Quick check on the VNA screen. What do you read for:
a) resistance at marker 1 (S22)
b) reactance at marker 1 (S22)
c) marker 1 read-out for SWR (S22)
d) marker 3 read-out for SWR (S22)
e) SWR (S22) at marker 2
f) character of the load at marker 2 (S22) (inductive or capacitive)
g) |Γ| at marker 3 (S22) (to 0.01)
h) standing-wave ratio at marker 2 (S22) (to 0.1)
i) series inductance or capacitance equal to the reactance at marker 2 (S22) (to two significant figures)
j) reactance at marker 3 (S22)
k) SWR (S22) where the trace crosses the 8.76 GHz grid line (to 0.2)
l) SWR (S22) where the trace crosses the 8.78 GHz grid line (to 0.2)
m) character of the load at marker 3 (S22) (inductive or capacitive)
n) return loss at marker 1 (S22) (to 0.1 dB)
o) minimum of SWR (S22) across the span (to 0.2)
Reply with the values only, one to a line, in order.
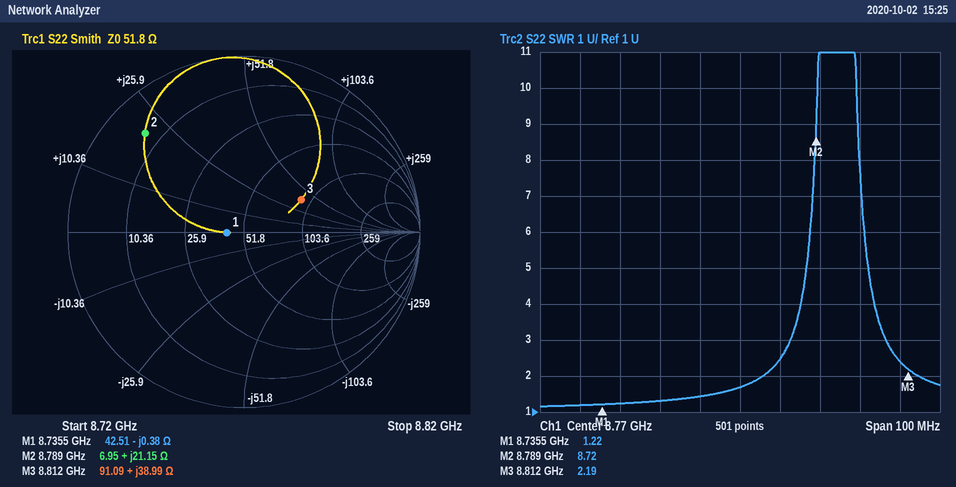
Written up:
42.51 Ω
-0.38 Ω
1.22
2.19
8.72
inductive
0.37
8.7
380 pH
+38.99 Ω
1.4
2.4
inductive
20.1 dB
1.2
